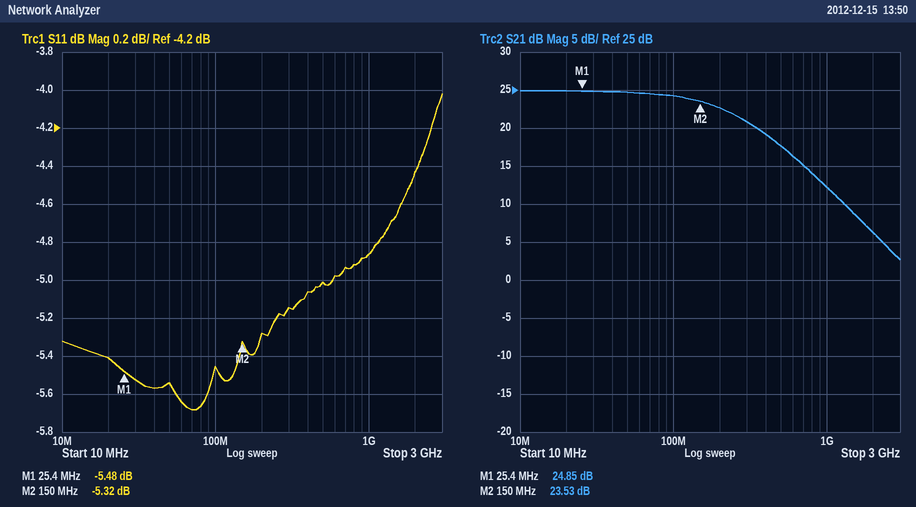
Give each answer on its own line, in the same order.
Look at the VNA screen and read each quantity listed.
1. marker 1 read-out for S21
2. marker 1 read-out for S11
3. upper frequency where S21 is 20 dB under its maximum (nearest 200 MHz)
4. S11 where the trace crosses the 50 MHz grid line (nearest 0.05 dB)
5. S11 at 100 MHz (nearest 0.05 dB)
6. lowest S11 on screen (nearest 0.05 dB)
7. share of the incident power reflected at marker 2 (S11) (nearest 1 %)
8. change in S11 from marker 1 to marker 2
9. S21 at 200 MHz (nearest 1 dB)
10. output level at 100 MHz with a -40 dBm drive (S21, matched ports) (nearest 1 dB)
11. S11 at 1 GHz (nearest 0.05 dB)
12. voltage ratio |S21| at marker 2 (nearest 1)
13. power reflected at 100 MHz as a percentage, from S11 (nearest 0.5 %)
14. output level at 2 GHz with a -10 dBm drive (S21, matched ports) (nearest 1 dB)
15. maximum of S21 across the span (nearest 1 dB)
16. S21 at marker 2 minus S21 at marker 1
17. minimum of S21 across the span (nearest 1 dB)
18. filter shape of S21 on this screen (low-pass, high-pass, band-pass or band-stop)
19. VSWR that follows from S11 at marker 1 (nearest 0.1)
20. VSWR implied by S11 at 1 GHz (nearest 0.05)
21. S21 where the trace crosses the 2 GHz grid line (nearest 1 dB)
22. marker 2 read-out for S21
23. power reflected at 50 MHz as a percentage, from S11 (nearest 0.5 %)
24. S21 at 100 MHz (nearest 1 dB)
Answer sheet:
24.85 dB
-5.48 dB
2.4 GHz
-5.55 dB
-5.45 dB
-5.70 dB
29 %
0.16 dB
23 dB
-16 dBm
-4.85 dB
15
28.5 %
-4 dBm
25 dB
-1.32 dB
3 dB
low-pass
3.3
3.65
6 dB
23.53 dB
28.0 %
24 dB
